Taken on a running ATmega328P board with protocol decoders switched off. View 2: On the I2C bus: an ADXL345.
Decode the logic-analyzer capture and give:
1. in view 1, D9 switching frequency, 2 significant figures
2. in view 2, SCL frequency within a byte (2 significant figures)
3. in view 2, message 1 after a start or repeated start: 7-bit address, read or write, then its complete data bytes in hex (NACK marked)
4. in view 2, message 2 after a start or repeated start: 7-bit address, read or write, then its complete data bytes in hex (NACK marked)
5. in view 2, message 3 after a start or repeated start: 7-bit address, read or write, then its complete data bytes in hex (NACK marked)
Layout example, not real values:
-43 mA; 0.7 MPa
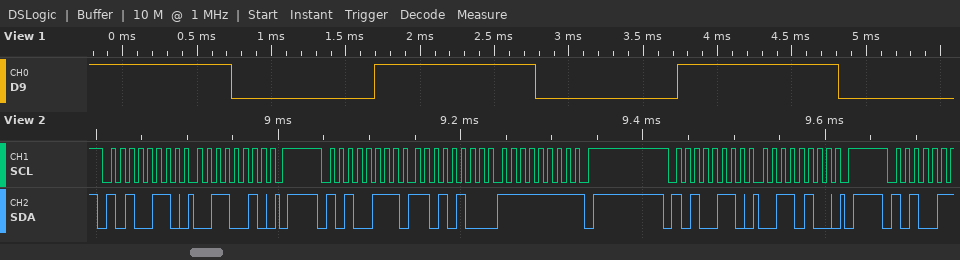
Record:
490 Hz; 100 kHz; 0x53 write: 32; 0x53 read: D4 FF NACK; 0x53 write: 34
